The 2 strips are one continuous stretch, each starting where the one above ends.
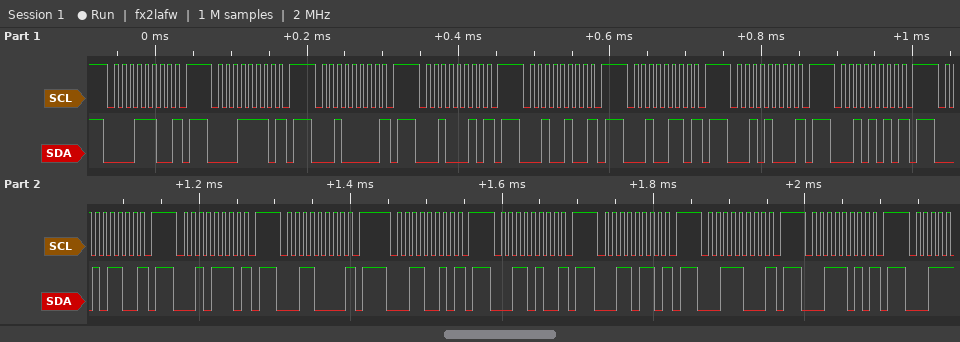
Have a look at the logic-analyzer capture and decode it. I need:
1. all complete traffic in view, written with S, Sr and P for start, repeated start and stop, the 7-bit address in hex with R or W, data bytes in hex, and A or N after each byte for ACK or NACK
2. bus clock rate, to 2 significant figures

S 0EW N P S 0FW N P S 10W N P S 11W N P S 12W N P S 13W N P S 14W N P S 15W N P S 16W N P S 17W N P S 18W N P S 19W N P S 1AW N P S 1BW N P S 1CW N P S 1DW N P
100 kHz
